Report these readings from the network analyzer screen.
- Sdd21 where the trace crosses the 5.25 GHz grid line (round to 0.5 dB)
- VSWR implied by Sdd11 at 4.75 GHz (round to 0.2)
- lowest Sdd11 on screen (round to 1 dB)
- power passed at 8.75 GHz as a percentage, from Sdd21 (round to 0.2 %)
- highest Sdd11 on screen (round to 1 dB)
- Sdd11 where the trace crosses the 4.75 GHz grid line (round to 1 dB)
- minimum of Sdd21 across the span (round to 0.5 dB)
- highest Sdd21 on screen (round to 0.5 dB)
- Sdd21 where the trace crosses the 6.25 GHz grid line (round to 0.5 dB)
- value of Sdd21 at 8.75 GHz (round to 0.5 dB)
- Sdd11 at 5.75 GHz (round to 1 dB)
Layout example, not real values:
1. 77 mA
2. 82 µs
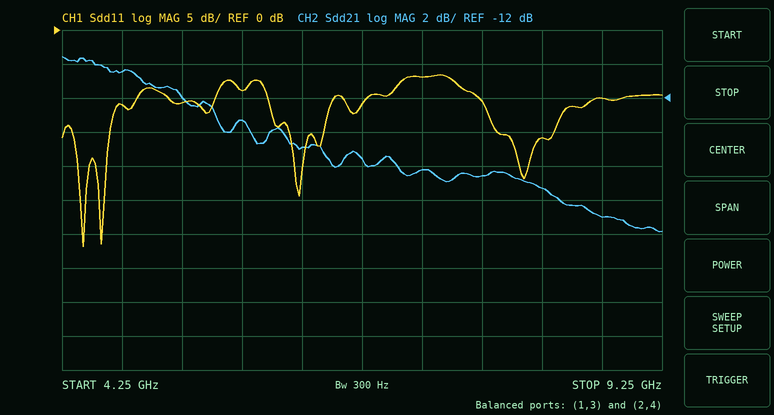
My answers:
1. -12.0 dB
2. 1.8
3. -32 dB
4. 1.2 %
5. -7 dB
6. -11 dB
7. -20.0 dB
8. -9.5 dB
9. -15.0 dB
10. -19.0 dB
11. -9 dB
